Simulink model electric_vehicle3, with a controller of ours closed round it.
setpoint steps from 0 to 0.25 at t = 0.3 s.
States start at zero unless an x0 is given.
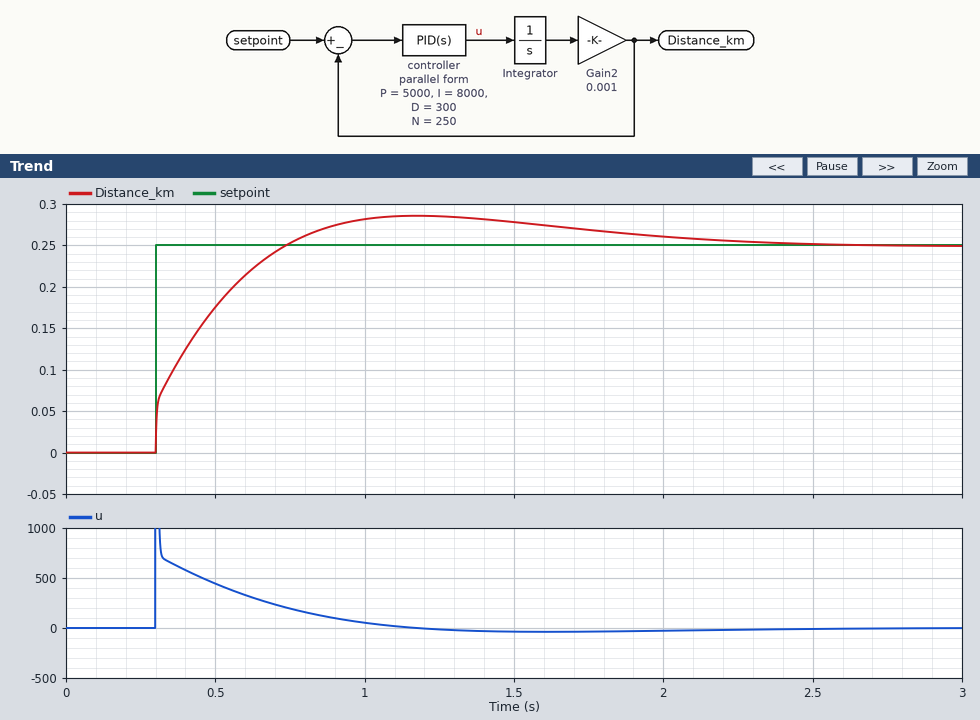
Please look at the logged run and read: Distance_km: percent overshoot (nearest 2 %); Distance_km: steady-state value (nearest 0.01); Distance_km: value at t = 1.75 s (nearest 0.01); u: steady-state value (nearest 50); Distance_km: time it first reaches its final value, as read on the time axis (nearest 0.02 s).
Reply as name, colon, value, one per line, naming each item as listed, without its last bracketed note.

Distance_km: percent overshoot: 14 %
Distance_km: steady-state value: 0.25
Distance_km: value at t = 1.75 s: 0.27
u: steady-state value: 0
Distance_km: time it first reaches its final value, as read on the time axis: 0.74 s
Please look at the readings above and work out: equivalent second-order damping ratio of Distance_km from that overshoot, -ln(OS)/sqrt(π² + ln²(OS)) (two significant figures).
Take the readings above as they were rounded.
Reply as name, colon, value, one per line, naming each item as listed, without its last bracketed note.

equivalent second-order damping ratio of Distance_km from that overshoot, -ln(OS)/sqrt(π² + ln²(OS)): 0.53
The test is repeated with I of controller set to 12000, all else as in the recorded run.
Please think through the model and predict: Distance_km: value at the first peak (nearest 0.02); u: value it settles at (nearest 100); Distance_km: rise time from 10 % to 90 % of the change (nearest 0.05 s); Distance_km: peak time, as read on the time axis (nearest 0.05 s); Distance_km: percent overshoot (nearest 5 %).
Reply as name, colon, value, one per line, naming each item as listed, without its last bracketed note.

Distance_km: value at the first peak: 0.30
u: value it settles at: 0
Distance_km: rise time from 10 % to 90 % of the change: 0.30 s
Distance_km: peak time, as read on the time axis: 1.05 s
Distance_km: percent overshoot: 20 %
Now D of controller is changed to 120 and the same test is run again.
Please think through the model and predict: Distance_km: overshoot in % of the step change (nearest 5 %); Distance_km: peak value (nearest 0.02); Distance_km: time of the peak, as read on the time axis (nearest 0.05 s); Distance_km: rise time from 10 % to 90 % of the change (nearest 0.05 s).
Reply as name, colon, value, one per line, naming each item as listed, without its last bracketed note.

Distance_km: overshoot in % of the step change: 15 %
Distance_km: peak value: 0.28
Distance_km: time of the peak, as read on the time axis: 1.10 s
Distance_km: rise time from 10 % to 90 % of the change: 0.30 s
